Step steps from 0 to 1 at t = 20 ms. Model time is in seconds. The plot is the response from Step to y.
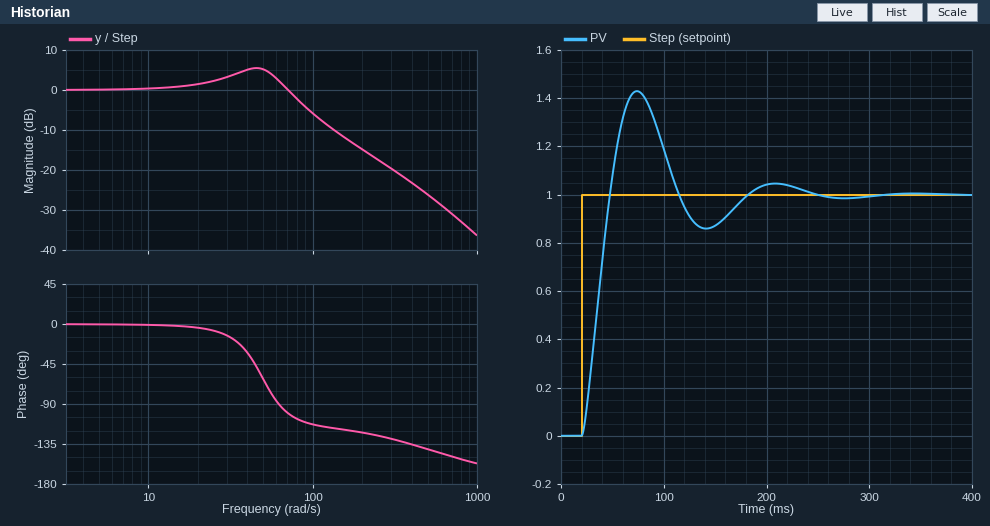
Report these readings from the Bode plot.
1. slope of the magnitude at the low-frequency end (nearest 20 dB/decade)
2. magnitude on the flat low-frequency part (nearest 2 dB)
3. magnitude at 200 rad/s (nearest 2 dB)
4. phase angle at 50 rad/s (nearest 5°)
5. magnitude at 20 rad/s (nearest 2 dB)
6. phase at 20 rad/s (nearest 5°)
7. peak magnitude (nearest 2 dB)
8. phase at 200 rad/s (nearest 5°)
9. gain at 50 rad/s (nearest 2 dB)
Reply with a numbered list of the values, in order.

1. 0 dB/decade
2. 0 dB
3. -14 dB
4. -60°
5. 2 dB
6. -5°
7. 6 dB
8. -120°
9. 6 dB
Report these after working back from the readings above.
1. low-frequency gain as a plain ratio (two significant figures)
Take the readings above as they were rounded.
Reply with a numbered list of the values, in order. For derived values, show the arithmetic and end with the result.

1. 10^(0 / 20) = 1.0
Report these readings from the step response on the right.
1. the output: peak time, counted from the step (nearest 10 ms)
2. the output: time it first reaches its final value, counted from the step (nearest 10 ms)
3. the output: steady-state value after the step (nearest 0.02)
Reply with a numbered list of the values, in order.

1. 50 ms
2. 30 ms
3. 1.00
